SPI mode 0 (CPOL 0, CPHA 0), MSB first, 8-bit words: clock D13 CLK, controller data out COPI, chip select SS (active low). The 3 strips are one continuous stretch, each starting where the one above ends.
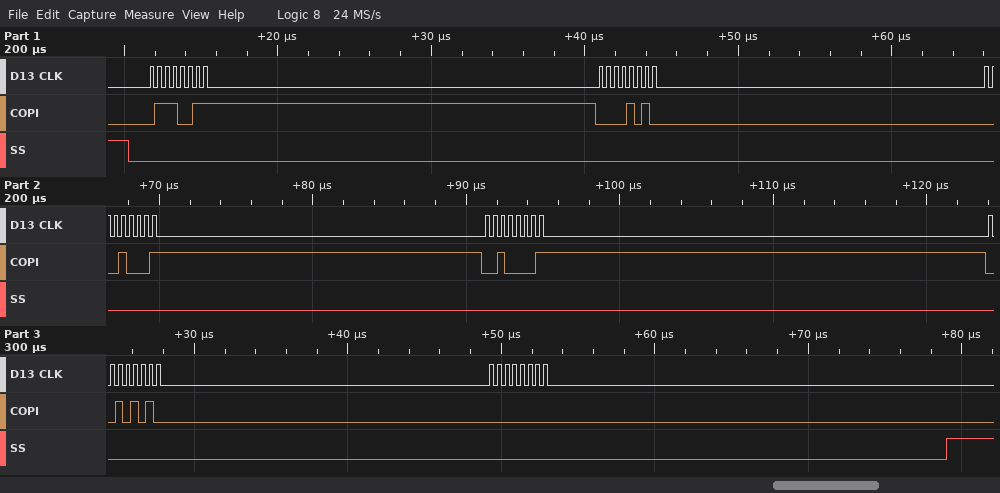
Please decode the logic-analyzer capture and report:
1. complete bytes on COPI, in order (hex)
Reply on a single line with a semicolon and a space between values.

73 0A 11 21 2A 00
